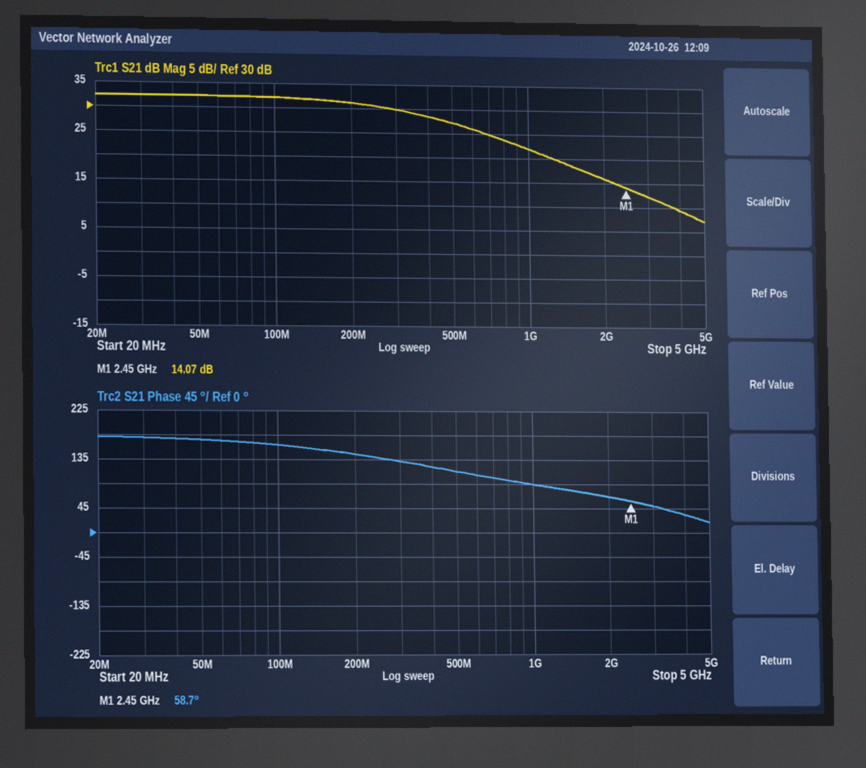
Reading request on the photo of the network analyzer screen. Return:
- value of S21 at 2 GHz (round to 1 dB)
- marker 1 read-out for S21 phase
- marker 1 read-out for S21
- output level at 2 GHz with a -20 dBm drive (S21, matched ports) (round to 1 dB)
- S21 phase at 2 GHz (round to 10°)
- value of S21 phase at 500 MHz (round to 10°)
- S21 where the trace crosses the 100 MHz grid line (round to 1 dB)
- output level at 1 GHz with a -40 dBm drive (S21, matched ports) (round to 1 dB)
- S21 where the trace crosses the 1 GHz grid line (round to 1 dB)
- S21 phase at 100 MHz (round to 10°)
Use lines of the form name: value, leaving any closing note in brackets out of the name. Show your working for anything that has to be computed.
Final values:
value of S21 at 2 GHz: 16 dB
marker 1 read-out for S21 phase: 58.7°
marker 1 read-out for S21: 14.07 dB
output level at 2 GHz with a -20 dBm drive (S21, matched ports): -20 dBm + (16 dB) = -4 dBm
S21 phase at 2 GHz: 70°
value of S21 phase at 500 MHz: 110°
S21 where the trace crosses the 100 MHz grid line: 32 dB
output level at 1 GHz with a -40 dBm drive (S21, matched ports): -40 dBm + (22 dB) = -18 dBm
S21 where the trace crosses the 1 GHz grid line: 22 dB
S21 phase at 100 MHz: 160°
